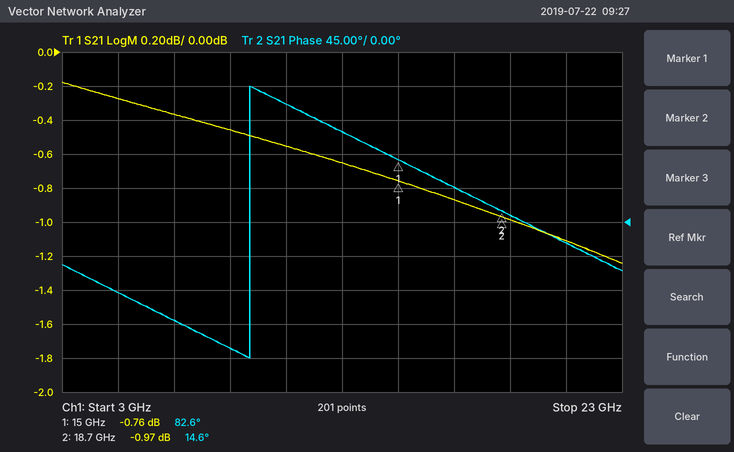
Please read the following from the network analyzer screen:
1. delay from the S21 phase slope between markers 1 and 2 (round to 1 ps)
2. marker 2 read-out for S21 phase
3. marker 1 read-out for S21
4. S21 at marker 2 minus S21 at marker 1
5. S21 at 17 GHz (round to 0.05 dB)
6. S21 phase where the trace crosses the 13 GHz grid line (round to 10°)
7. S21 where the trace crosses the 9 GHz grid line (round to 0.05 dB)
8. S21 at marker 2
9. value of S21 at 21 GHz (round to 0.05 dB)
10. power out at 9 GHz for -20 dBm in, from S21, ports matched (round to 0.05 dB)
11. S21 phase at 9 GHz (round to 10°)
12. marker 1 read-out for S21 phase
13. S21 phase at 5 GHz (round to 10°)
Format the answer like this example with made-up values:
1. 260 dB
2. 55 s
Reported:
1. 51 ps
2. 14.6°
3. -0.76 dB
4. -0.21 dB
5. -0.85 dB
6. 120°
7. -0.45 dB
8. -0.97 dB
9. -1.10 dB
10. -20.45 dBm
11. -170°
12. 82.6°
13. -90°
